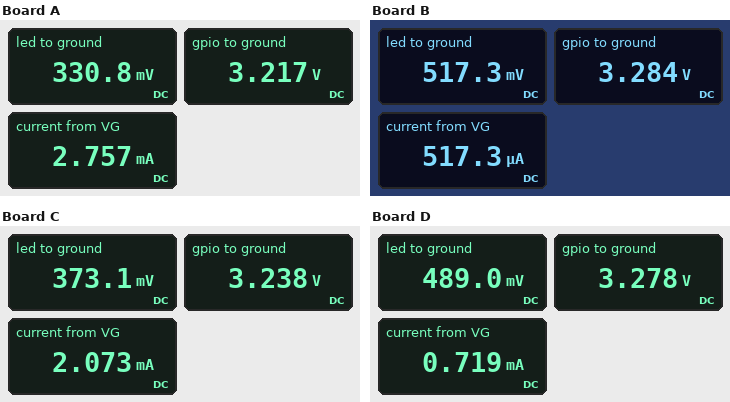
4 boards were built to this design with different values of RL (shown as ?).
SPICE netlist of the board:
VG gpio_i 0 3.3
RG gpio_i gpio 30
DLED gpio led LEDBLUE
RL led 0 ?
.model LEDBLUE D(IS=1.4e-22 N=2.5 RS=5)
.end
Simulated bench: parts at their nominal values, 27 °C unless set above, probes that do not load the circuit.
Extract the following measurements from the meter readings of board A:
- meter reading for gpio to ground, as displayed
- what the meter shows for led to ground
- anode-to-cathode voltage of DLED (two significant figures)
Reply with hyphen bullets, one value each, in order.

- 3.217 V
- 330.8 mV
- 2.9 V
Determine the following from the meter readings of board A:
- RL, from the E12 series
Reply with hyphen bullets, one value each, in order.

- 120 Ω
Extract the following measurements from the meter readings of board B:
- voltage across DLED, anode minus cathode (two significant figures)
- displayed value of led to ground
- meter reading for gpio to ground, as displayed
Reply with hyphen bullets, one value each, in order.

- 2.8 V
- 517.3 mV
- 3.284 V
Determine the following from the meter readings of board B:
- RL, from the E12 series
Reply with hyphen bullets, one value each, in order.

- 1 kΩ
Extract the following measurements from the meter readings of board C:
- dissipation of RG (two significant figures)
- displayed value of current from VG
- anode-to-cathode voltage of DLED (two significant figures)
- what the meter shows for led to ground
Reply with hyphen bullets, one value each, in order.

- 130 µW
- 2.073 mA
- 2.9 V
- 373.1 mV
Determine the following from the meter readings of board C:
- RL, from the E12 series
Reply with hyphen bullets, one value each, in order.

- 180 Ω
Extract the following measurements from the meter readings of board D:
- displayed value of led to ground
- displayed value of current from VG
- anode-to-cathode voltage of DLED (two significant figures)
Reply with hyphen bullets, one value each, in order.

- 489.0 mV
- 0.719 mA
- 2.8 V
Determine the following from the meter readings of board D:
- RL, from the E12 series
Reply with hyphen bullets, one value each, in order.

- 680 Ω
